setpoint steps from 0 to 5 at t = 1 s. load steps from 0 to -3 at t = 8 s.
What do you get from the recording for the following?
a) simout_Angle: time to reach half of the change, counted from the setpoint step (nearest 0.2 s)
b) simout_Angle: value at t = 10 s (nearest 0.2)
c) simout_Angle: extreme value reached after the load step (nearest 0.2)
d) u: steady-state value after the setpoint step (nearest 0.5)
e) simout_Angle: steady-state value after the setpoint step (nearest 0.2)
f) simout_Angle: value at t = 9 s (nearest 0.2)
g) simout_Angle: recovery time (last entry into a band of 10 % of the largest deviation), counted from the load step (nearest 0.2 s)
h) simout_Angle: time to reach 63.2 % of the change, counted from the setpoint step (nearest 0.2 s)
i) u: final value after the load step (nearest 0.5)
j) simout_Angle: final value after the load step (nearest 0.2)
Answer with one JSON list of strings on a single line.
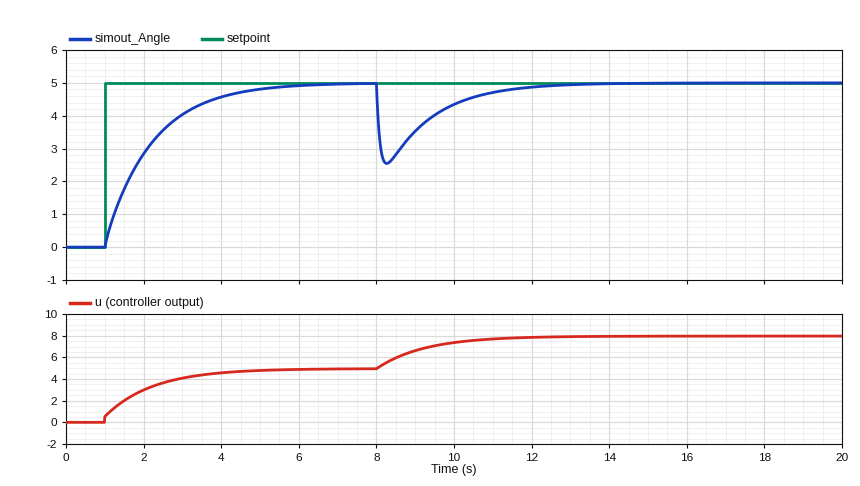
["0.8 s", "4.4", "2.6", "5.0", "5.0", "3.6", "3.2 s", "1.2 s", "8.0", "5.0"]
